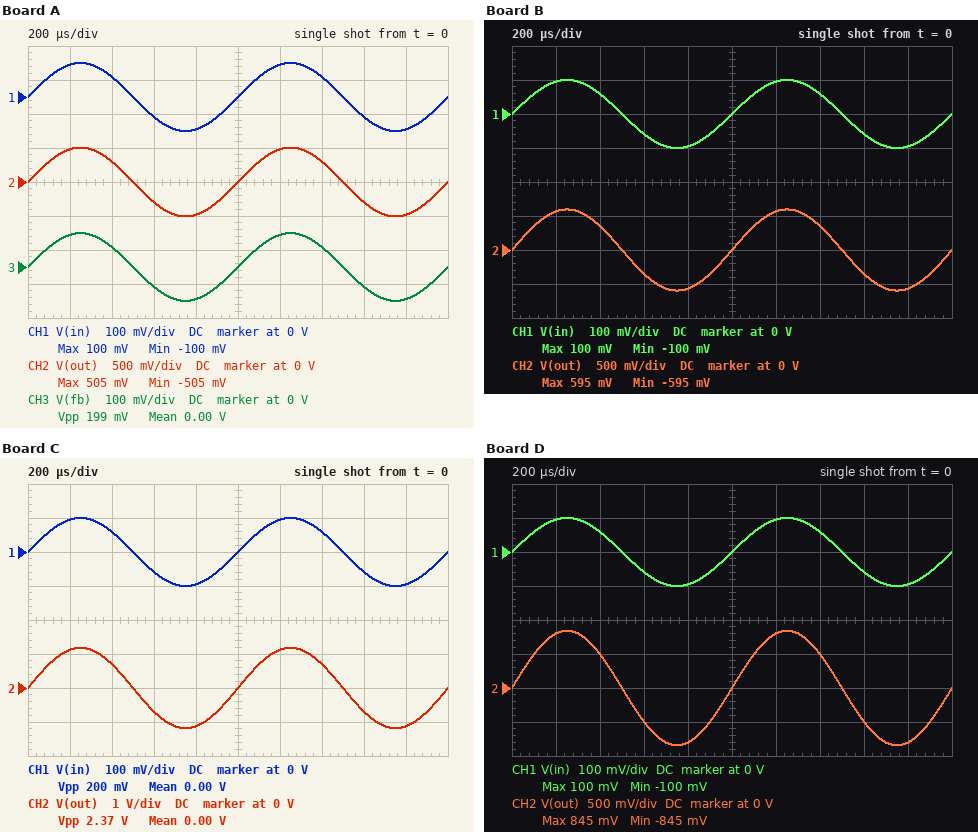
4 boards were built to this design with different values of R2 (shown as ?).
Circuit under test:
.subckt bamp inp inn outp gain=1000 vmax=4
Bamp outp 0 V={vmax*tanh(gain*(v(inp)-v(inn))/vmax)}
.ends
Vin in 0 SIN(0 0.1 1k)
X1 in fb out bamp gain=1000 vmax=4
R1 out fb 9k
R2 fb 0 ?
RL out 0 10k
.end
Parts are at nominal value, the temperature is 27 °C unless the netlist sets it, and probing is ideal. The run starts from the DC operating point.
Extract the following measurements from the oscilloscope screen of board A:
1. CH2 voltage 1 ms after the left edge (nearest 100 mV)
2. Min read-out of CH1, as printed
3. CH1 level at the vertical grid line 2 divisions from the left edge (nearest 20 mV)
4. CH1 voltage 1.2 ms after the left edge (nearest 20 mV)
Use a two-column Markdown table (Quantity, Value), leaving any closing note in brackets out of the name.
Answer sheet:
| Quantity | Value |
|---|---|
| CH2 voltage 1 ms after the left edge | 0 V |
| Min read-out of CH1, as printed | -100 mV |
| CH1 level at the vertical grid line 2 divisions from the left edge | 60 mV |
| CH1 voltage 1.2 ms after the left edge | 100 mV |
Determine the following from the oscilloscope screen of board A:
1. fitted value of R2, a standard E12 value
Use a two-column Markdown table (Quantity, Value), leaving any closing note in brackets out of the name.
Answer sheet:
| Quantity | Value |
|---|---|
| fitted value of R2, a standard E12 value | 2.2 kΩ |
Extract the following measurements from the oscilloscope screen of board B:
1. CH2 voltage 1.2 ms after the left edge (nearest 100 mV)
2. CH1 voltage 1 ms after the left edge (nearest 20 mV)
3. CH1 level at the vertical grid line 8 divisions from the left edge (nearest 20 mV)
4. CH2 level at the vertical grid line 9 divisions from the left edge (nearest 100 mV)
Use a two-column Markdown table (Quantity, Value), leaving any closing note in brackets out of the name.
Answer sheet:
| Quantity | Value |
|---|---|
| CH2 voltage 1.2 ms after the left edge | 600 mV |
| CH1 voltage 1 ms after the left edge | 0 V |
| CH1 level at the vertical grid line 8 divisions from the left edge | -60 mV |
| CH2 level at the vertical grid line 9 divisions from the left edge | -600 mV |
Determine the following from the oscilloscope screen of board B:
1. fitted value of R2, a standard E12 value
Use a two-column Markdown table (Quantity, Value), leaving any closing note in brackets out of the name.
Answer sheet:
| Quantity | Value |
|---|---|
| fitted value of R2, a standard E12 value | 1.8 kΩ |
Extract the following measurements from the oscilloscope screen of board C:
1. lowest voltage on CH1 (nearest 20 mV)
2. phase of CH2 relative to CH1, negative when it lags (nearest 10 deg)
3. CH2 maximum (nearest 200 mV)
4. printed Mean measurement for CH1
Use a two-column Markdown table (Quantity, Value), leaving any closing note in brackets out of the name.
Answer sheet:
| Quantity | Value |
|---|---|
| lowest voltage on CH1 | -100 mV |
| phase of CH2 relative to CH1, negative when it lags | 0 deg |
| CH2 maximum | 1.2 V |
| printed Mean measurement for CH1 | 0.00 V |
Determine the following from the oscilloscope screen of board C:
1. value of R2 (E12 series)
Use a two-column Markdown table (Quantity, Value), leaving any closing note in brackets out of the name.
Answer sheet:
| Quantity | Value |
|---|---|
| value of R2 | 820 Ω |
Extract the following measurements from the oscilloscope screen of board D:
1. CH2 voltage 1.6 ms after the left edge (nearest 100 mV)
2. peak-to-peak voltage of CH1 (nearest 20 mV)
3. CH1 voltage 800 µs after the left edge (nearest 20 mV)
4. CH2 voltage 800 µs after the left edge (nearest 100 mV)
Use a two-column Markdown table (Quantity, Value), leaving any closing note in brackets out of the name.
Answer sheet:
| Quantity | Value |
|---|---|
| CH2 voltage 1.6 ms after the left edge | -500 mV |
| peak-to-peak voltage of CH1 | 200 mV |
| CH1 voltage 800 µs after the left edge | -100 mV |
| CH2 voltage 800 µs after the left edge | -800 mV |
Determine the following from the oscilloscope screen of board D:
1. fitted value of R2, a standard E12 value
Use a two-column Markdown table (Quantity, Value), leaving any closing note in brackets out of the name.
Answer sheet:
| Quantity | Value |
|---|---|
| fitted value of R2, a standard E12 value | 1.2 kΩ |
